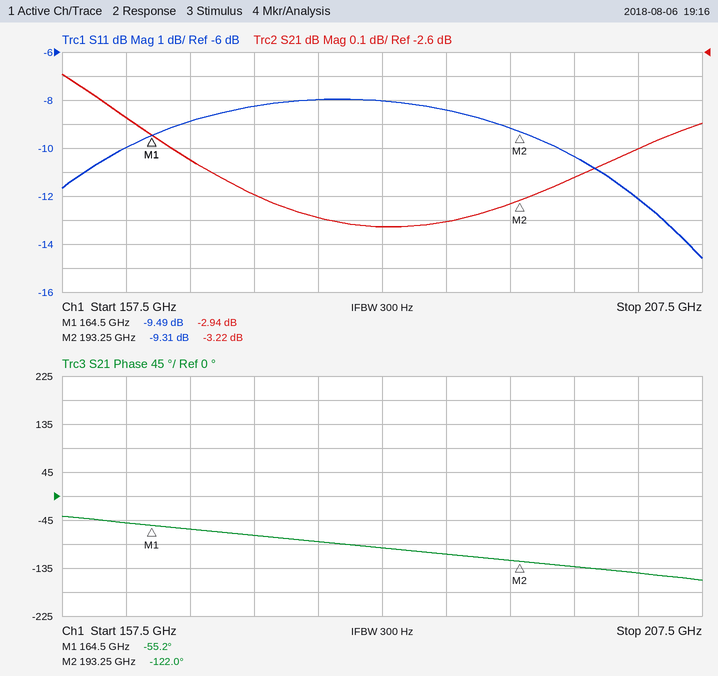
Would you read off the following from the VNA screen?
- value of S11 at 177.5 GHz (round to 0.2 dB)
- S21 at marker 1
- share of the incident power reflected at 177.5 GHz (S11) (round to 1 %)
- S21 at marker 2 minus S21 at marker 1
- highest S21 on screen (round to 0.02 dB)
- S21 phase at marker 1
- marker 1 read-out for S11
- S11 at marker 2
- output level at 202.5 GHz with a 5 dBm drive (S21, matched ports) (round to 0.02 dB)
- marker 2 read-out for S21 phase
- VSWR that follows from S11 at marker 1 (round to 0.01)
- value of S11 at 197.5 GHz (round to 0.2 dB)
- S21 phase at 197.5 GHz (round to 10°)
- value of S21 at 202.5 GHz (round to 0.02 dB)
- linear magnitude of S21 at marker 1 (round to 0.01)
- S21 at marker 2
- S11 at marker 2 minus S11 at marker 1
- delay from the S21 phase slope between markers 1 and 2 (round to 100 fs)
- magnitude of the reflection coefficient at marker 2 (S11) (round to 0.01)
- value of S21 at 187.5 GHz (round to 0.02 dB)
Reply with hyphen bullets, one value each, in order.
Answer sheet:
- -8.0 dB
- -2.94 dB
- 16 %
- -0.28 dB
- -2.70 dB
- -55.2°
- -9.49 dB
- -9.31 dB
- 2.00 dBm
- -122.0°
- 2.01
- -10.4 dB
- -130°
- -3.00 dB
- 0.71
- -3.22 dB
- 0.18 dB
- 6.5 ps
- 0.34
- -3.30 dB
